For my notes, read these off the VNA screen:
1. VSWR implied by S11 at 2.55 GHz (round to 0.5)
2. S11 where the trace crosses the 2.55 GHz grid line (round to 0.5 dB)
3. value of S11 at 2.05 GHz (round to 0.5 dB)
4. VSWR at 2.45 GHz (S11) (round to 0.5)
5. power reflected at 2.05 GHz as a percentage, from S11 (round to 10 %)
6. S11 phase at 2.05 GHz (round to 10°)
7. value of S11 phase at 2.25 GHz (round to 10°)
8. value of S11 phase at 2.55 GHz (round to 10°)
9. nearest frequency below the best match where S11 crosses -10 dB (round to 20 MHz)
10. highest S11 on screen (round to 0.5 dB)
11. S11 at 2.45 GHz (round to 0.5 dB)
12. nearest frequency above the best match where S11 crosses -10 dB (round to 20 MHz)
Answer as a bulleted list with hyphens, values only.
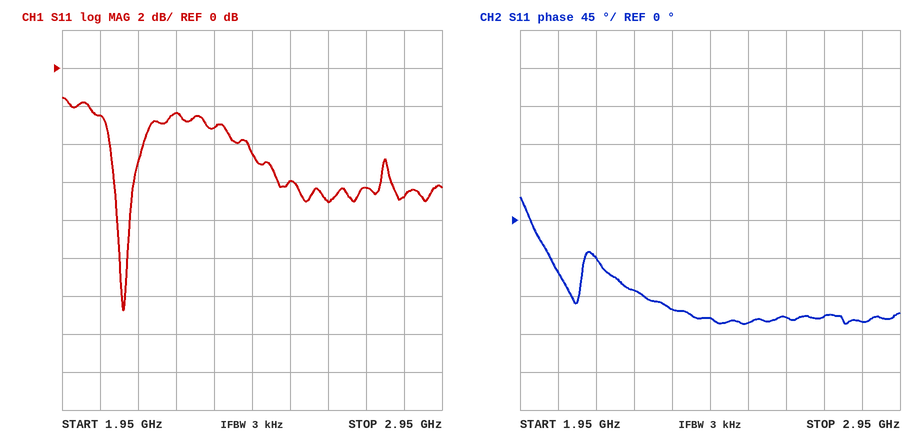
- 3.0
- -6.0 dB
- -2.5 dB
- 4.0
- 60 %
- -60°
- -80°
- -120°
- 2.10 GHz
- -1.5 dB
- -4.5 dB
- 2.12 GHz
